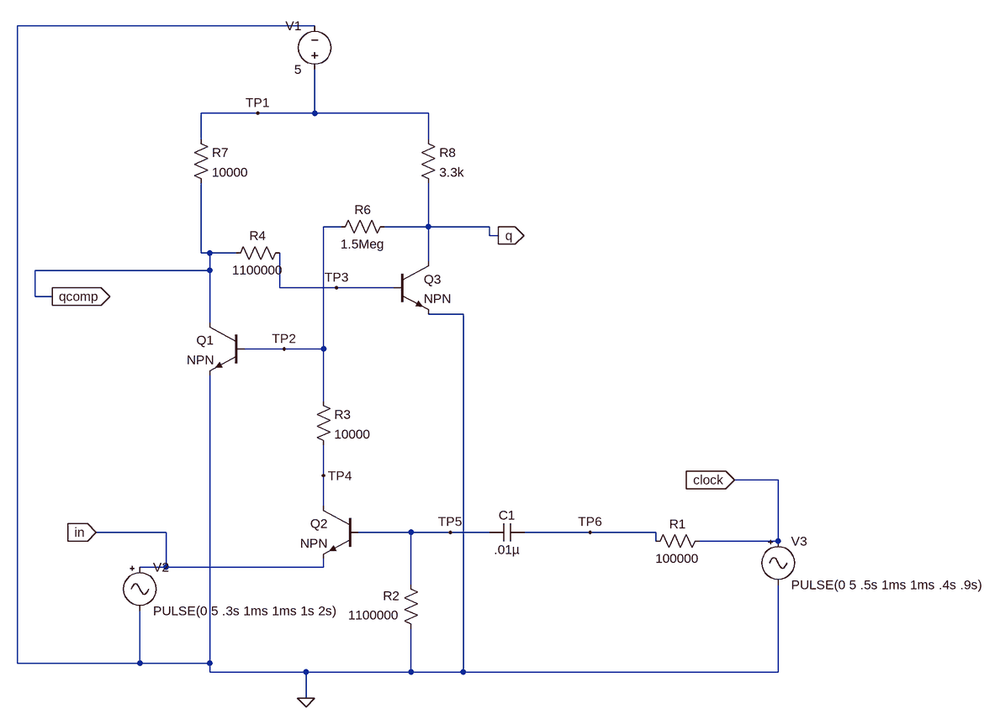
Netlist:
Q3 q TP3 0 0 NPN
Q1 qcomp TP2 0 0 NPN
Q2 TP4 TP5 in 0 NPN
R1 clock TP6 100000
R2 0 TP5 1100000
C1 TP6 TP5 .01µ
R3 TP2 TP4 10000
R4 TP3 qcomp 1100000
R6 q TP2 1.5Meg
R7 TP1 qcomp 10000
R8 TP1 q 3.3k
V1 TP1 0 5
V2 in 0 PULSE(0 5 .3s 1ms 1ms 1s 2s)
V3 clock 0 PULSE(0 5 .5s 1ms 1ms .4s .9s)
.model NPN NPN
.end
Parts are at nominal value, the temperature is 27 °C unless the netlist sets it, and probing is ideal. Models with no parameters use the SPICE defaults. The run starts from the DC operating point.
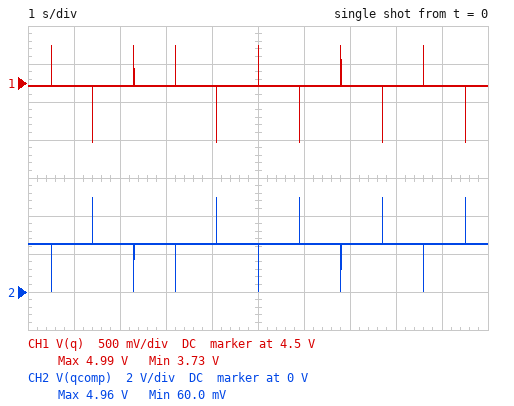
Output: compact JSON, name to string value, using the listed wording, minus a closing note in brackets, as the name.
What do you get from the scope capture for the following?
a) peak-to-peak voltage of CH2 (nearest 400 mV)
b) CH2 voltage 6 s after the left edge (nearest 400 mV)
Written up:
{"peak-to-peak voltage of CH2": "4.8 V", "CH2 voltage 6 s after the left edge": "2.4 V"}
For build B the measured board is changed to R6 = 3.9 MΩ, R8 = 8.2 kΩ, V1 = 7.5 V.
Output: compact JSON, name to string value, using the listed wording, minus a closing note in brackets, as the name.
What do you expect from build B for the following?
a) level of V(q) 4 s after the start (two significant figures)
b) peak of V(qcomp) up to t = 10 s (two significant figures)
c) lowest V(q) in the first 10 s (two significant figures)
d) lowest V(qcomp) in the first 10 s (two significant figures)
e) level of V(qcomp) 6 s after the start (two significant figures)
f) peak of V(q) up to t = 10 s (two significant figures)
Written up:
{"level of V(q) 4 s after the start": "2.9 V", "peak of V(qcomp) up to t = 10 s": "7.4 V", "lowest V(q) in the first 10 s": "2.5 V", "lowest V(qcomp) in the first 10 s": "81 mV", "level of V(qcomp) 6 s after the start": "6.9 V", "peak of V(q) up to t = 10 s": "7.5 V"}
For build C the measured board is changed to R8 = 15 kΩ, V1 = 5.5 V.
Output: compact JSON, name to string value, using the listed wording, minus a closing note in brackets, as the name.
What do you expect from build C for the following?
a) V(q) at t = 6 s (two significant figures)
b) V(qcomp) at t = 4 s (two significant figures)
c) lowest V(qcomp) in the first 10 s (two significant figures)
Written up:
{"V(q) at t = 6 s": "160 mV", "V(qcomp) at t = 4 s": "5.5 V", "lowest V(qcomp) in the first 10 s": "72 mV"}
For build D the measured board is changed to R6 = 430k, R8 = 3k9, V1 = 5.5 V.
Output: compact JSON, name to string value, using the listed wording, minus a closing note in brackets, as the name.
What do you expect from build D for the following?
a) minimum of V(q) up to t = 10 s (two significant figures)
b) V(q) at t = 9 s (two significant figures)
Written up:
{"minimum of V(q) up to t = 10 s": "3.8 V", "V(q) at t = 9 s": "5.5 V"}
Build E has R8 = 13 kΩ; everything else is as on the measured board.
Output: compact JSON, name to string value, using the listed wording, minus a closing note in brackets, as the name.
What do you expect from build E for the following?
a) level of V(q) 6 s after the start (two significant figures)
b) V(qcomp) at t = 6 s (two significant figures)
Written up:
{"level of V(q) 6 s after the start": "200 mV", "V(qcomp) at t = 6 s": "5.0 V"}
